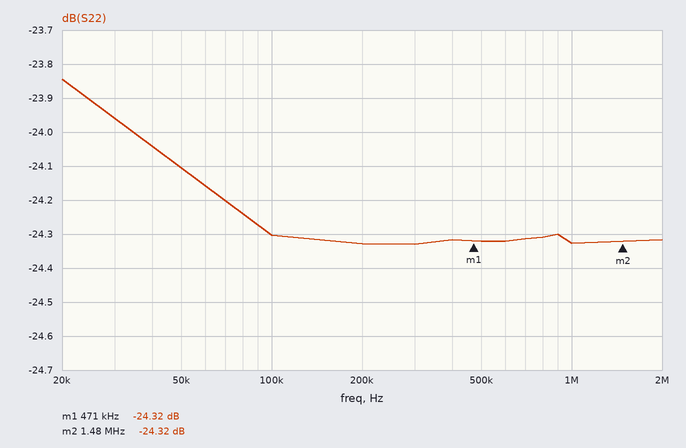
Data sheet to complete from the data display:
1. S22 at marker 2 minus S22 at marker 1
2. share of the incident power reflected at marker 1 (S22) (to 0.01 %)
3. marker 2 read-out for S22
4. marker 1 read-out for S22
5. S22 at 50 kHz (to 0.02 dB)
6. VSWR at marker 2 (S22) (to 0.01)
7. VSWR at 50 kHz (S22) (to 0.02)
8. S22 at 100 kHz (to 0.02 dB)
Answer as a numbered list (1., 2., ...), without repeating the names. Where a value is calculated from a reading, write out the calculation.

1. -24.32 − (-24.32) = 0.00 dB
2. 10^(-24.32/10) ≈ 0.37 %
3. -24.32 dB
4. -24.32 dB
5. -24.10 dB
6. (1 + 0.0608)/(1 − 0.0608) ≈ 1.13
7. |Γ| = 10^(-24.1/20) = 0.0624; VSWR = (1 + 0.0624)/(1 − 0.0624) ≈ 1.13, so 1.14 to the nearest 0.02
8. -24.30 dB
